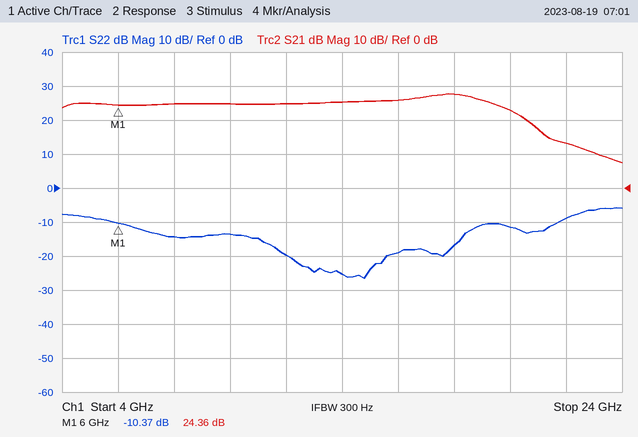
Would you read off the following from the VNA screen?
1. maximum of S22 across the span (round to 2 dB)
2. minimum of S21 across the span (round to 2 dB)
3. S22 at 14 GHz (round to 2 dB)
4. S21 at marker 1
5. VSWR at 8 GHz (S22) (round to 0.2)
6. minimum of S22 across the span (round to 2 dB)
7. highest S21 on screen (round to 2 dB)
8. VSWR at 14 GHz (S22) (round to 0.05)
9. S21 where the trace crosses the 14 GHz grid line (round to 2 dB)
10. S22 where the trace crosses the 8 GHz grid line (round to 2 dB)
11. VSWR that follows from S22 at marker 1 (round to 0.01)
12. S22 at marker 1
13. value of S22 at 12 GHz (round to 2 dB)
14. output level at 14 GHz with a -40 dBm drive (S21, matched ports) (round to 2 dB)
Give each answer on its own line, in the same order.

-6 dB
8 dB
-26 dB
24.36 dB
1.4
-26 dB
28 dB
1.10
26 dB
-14 dB
1.87
-10.37 dB
-20 dB
-14 dBm
